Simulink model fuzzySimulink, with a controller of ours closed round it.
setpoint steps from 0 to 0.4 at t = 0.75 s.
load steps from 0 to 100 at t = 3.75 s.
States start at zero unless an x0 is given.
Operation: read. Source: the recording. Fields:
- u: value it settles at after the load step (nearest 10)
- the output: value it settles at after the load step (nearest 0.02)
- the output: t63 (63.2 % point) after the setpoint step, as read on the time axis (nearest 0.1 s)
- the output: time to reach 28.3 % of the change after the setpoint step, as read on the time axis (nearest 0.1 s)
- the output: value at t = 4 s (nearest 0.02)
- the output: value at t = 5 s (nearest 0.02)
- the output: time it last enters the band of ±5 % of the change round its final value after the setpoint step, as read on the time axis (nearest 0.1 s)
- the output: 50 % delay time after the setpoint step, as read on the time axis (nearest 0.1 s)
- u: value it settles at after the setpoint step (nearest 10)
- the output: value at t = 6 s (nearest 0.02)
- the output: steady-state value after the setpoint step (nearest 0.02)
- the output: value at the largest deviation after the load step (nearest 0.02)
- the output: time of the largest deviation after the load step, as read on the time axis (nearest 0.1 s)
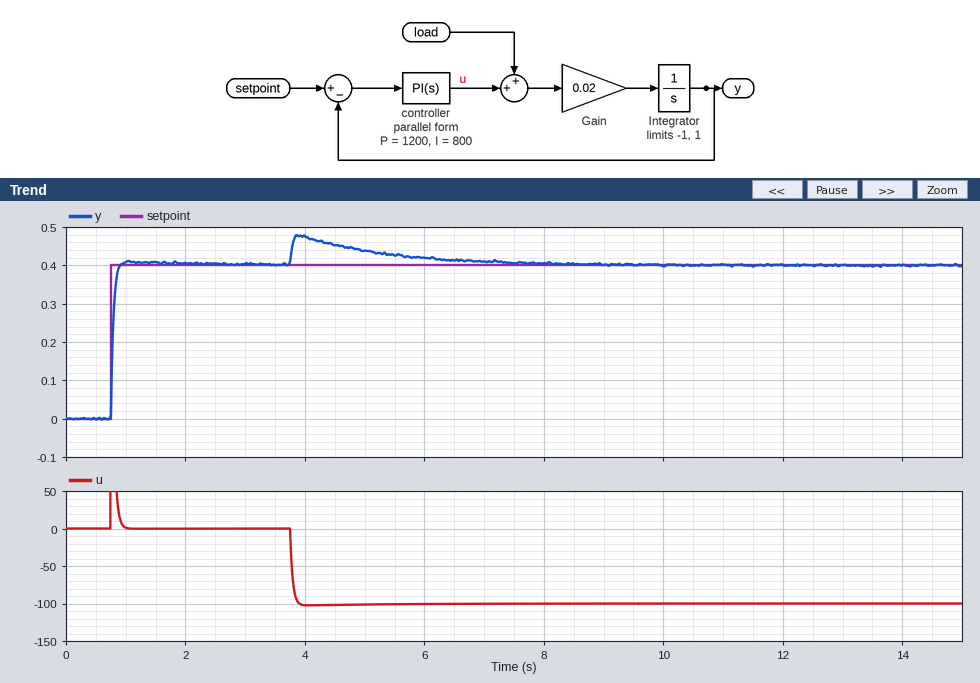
-100
0.40
0.8 s
0.8 s
0.48
0.44
0.9 s
0.8 s
0
0.42
0.40
0.48
3.9 s
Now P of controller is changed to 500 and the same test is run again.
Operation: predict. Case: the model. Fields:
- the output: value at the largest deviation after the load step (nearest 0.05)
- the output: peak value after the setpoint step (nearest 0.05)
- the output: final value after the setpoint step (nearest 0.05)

0.55
0.45
0.40
